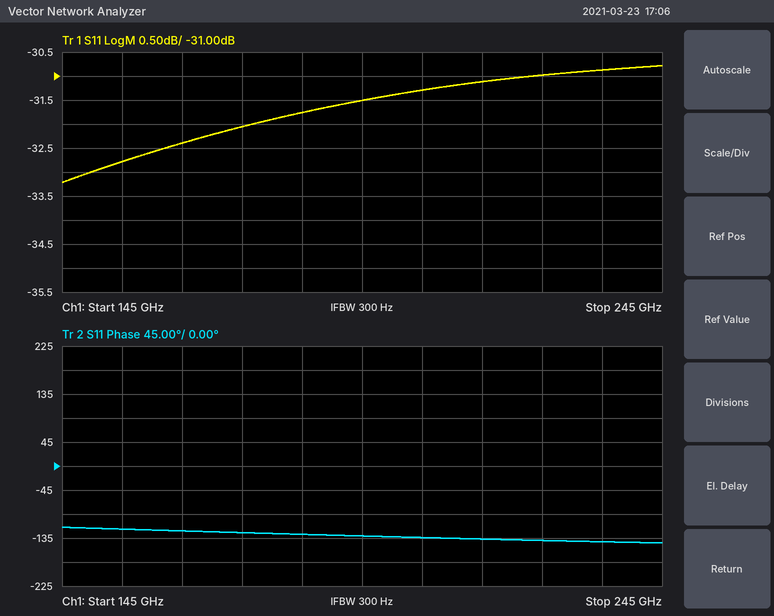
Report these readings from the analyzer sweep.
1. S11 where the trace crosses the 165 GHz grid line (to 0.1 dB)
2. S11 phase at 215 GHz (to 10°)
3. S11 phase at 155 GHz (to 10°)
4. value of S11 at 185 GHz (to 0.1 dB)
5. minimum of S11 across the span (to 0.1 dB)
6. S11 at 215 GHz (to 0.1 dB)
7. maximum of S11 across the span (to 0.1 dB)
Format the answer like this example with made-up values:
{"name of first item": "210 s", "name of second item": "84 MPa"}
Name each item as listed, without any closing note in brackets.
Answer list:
{"S11 where the trace crosses the 165 GHz grid line": "-32.4 dB", "S11 phase at 215 GHz": "-140°", "S11 phase at 155 GHz": "-120°", "value of S11 at 185 GHz": "-31.8 dB", "minimum of S11 across the span": "-33.2 dB", "S11 at 215 GHz": "-31.1 dB", "maximum of S11 across the span": "-30.8 dB"}
